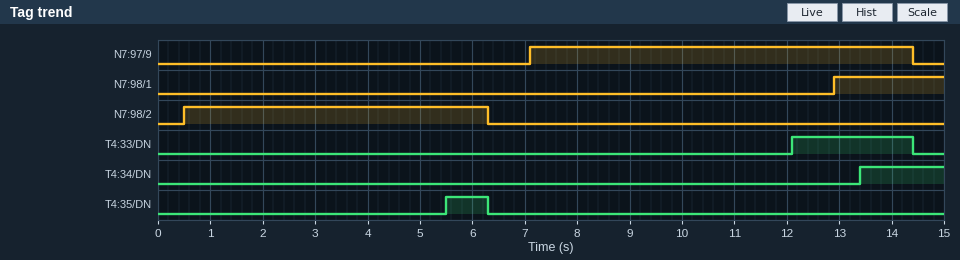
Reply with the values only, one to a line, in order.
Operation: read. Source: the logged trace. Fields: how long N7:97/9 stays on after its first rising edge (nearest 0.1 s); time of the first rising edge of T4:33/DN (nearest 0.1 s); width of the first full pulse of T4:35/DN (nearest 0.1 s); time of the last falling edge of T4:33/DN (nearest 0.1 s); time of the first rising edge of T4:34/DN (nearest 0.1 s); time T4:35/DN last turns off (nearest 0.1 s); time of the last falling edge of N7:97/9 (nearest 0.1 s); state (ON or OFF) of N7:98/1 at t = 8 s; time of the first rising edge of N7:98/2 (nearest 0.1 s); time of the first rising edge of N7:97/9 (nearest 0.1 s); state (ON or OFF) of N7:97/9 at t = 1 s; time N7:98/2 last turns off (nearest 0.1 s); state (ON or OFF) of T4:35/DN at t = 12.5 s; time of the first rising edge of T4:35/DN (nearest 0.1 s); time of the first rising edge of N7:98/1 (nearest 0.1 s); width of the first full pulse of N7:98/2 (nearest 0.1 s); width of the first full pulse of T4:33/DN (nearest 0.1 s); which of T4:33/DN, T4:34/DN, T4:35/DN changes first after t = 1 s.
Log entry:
7.3 s
12.1 s
0.8 s
14.4 s
13.4 s
6.3 s
14.4 s
OFF
0.5 s
7.1 s
OFF
6.3 s
OFF
5.5 s
12.9 s
5.8 s
2.3 s
T4:35/DN
